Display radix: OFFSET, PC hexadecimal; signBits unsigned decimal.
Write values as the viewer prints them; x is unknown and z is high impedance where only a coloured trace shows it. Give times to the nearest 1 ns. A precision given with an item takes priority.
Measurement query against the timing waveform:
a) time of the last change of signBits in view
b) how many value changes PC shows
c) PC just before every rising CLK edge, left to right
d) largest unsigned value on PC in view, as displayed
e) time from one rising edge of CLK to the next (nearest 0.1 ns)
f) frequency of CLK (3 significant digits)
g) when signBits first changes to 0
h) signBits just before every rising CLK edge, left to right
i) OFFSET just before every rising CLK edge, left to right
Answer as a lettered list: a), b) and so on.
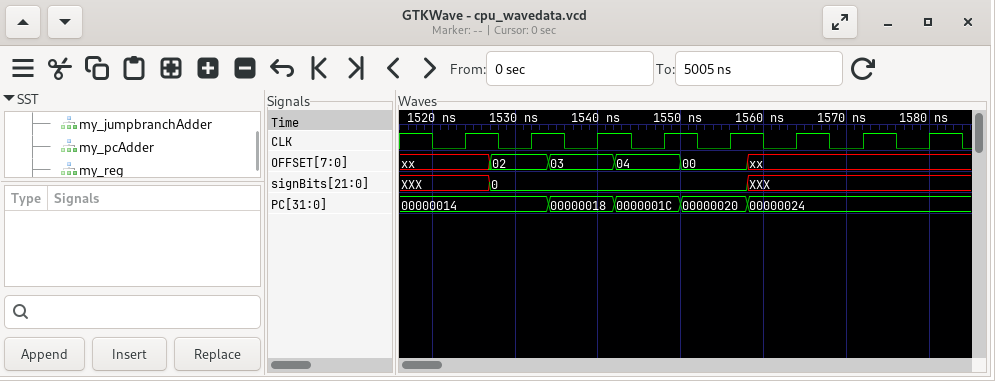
a) 1558 ns
b) 4
c) 00000014, 00000014, 00000018, 0000001C, 00000020, 00000024, 00000024, 00000024
d) 00000024
e) 8 ns
f) 125 MHz
g) 1527 ns
h) XXX, 0, 0, 0, 0, XXX, XXX, XXX
i) xx, 02, 03, 04, 00, xx, xx, xx
